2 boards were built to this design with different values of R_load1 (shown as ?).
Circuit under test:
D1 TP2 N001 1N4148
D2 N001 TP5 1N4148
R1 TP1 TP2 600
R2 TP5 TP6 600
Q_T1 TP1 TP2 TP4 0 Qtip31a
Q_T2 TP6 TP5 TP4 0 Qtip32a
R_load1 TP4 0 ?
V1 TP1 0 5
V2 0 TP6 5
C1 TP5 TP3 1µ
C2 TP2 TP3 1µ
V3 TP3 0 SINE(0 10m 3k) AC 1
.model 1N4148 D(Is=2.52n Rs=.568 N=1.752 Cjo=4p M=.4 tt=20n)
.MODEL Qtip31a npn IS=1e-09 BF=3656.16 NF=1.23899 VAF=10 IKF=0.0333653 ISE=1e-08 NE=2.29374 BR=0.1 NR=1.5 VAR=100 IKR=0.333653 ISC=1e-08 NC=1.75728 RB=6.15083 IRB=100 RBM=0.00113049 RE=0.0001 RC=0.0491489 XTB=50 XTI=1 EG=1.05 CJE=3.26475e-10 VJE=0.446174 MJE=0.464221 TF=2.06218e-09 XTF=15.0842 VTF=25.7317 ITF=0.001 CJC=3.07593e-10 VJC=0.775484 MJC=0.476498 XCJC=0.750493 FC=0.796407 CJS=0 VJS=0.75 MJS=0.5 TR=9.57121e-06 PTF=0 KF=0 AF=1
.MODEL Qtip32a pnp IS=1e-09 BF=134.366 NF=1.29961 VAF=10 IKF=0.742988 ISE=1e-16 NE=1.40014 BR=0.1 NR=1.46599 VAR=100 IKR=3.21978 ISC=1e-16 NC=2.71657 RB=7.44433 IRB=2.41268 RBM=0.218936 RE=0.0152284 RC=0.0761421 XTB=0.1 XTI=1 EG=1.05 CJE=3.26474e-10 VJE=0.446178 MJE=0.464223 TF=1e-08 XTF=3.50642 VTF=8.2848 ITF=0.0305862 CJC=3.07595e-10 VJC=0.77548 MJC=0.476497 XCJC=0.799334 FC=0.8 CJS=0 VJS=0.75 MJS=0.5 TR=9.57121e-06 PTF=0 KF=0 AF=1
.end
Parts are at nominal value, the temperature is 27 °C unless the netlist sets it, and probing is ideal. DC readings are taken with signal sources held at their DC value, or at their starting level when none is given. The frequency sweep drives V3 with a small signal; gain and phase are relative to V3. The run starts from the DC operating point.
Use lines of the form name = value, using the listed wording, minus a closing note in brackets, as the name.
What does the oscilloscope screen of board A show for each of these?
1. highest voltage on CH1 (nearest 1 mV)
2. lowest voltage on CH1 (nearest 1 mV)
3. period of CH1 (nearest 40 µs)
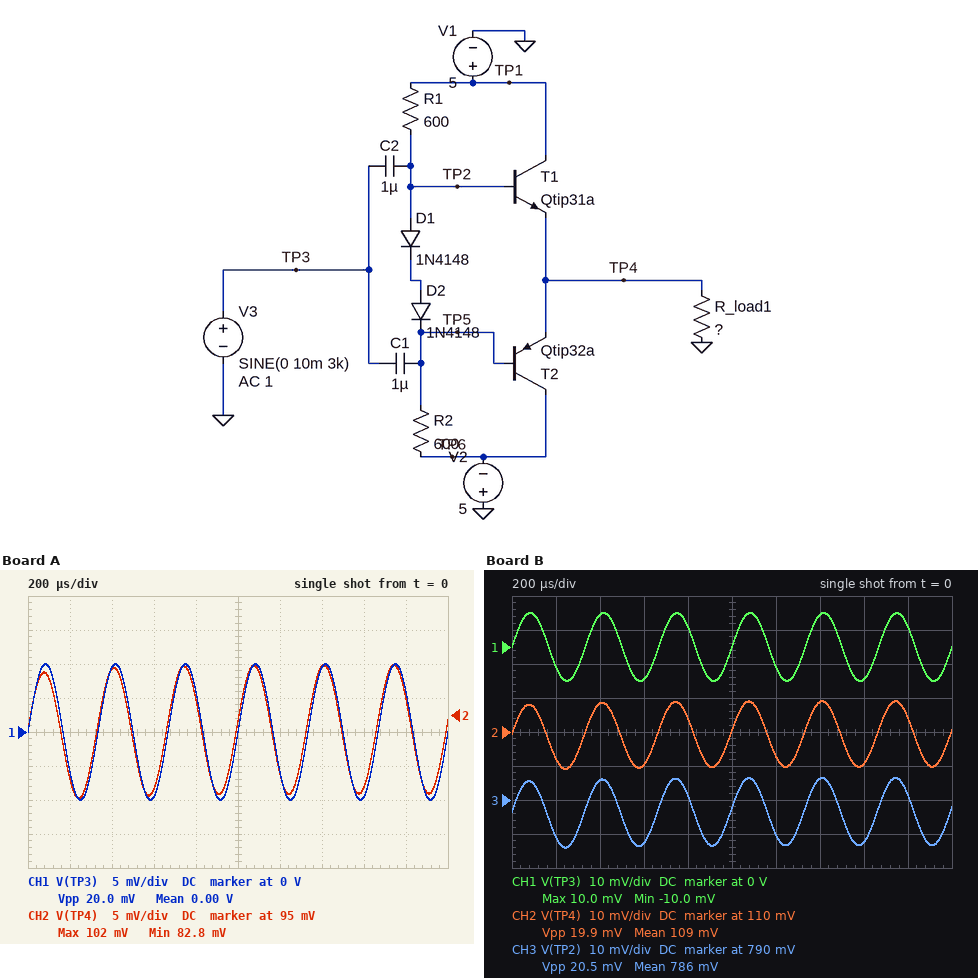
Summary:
highest voltage on CH1 = 10 mV
lowest voltage on CH1 = -10 mV
period of CH1 = 320 µs
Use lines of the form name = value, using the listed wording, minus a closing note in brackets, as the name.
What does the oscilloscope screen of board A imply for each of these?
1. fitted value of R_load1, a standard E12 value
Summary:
fitted value of R_load1, a standard E12 value = 3.3 Ω
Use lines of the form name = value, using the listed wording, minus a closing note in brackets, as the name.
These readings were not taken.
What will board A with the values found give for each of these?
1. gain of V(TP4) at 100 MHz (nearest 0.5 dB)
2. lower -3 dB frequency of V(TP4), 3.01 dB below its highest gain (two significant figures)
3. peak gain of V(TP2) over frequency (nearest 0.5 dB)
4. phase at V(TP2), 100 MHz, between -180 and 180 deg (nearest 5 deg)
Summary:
gain of V(TP4) at 100 MHz = -6.5 dB
lower -3 dB frequency of V(TP4), 3.01 dB below its highest gain = 430 Hz
peak gain of V(TP2) over frequency = 0 dB
phase at V(TP2), 100 MHz, between -180 and 180 deg = 0 deg
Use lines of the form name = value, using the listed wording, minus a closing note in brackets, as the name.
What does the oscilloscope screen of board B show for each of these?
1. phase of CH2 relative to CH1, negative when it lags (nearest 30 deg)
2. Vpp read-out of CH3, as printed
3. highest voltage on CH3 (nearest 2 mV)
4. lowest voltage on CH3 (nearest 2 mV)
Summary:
phase of CH2 relative to CH1, negative when it lags = 0 deg
Vpp read-out of CH3, as printed = 20.5 mV
highest voltage on CH3 = 796 mV
lowest voltage on CH3 = 776 mV
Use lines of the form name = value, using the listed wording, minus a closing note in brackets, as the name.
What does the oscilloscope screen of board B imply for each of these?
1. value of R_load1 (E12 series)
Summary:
value of R_load1 = 5.6 Ω
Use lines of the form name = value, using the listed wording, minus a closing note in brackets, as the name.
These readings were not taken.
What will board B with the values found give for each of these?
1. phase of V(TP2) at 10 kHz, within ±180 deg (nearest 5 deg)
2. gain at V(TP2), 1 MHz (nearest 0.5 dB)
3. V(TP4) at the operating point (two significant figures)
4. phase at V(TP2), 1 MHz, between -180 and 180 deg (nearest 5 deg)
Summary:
phase of V(TP2) at 10 kHz, within ±180 deg = 0 deg
gain at V(TP2), 1 MHz = 0 dB
V(TP4) at the operating point = 110 mV
phase at V(TP2), 1 MHz, between -180 and 180 deg = 0 deg
